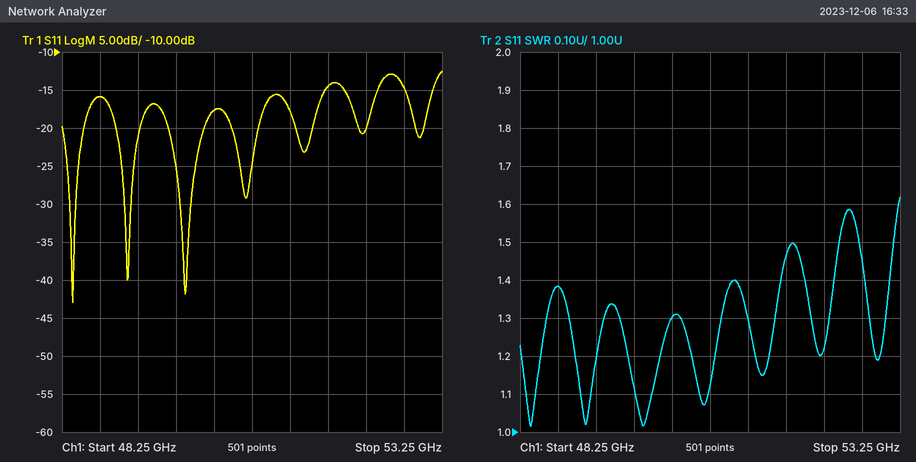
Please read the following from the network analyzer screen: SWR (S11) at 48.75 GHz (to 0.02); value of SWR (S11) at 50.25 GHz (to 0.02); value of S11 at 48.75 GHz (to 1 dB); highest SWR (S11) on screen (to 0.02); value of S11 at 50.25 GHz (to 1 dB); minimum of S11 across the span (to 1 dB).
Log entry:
1.38
1.30
-16 dB
1.62
-18 dB
-43 dB
